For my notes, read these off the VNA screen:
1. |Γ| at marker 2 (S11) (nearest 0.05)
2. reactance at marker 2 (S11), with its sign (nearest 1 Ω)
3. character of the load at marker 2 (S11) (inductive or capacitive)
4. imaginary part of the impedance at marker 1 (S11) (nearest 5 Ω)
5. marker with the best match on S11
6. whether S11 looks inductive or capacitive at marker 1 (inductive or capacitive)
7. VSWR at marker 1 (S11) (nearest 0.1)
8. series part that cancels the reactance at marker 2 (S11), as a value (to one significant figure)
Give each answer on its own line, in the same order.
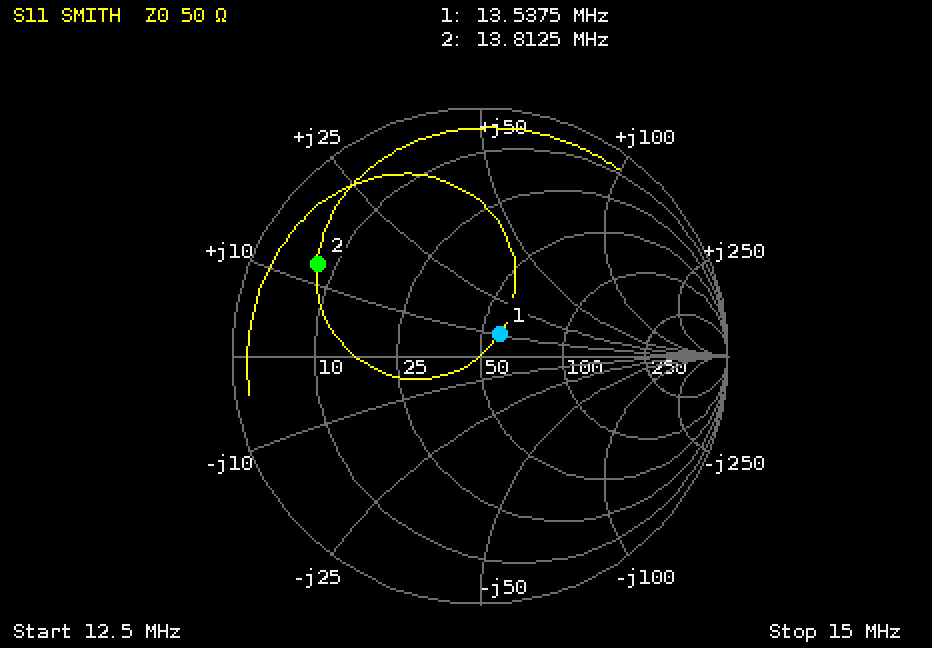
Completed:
0.75
+13 Ω
inductive
+10 Ω
marker 1
inductive
1.3
900 pF
